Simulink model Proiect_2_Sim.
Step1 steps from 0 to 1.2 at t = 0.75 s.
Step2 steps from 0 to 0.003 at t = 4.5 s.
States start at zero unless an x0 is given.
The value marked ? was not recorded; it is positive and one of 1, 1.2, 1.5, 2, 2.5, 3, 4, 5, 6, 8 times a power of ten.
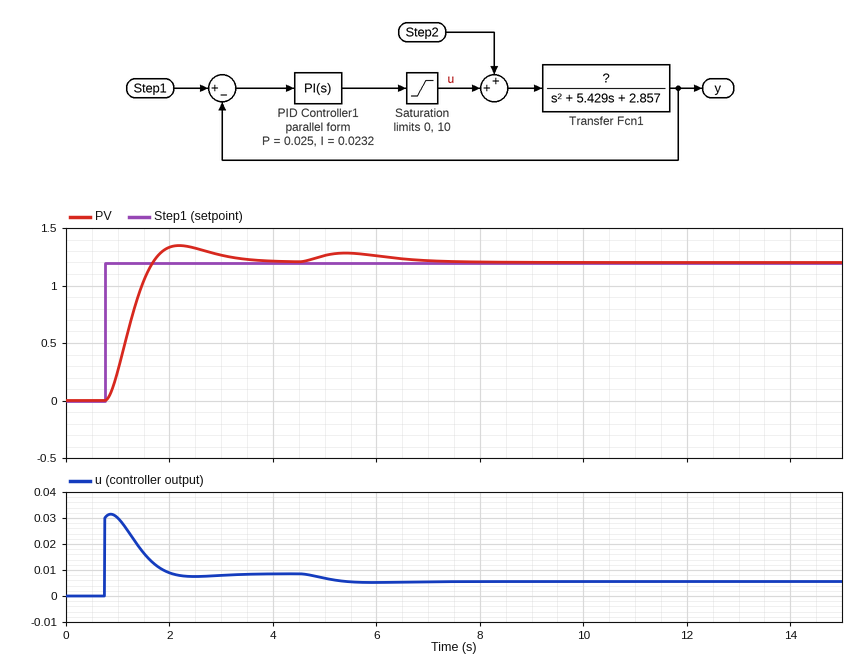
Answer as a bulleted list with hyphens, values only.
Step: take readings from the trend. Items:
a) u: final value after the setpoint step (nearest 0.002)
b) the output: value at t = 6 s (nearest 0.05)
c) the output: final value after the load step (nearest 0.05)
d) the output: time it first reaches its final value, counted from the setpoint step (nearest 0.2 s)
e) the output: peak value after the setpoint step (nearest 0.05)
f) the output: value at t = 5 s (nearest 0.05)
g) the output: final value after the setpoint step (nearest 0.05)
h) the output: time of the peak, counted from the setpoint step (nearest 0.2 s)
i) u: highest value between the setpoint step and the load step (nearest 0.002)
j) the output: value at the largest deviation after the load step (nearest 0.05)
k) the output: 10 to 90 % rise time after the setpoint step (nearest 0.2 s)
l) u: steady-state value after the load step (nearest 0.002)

- 0.008
- 1.25
- 1.20
- 1.0 s
- 1.35
- 1.25
- 1.20
- 1.4 s
- 0.032
- 1.30
- 0.6 s
- 0.006
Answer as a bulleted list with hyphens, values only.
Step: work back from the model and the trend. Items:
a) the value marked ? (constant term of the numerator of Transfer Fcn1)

- 400
